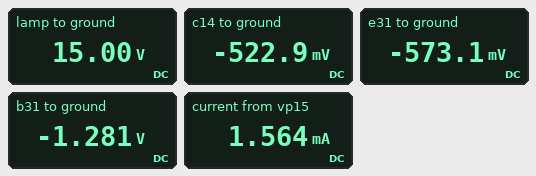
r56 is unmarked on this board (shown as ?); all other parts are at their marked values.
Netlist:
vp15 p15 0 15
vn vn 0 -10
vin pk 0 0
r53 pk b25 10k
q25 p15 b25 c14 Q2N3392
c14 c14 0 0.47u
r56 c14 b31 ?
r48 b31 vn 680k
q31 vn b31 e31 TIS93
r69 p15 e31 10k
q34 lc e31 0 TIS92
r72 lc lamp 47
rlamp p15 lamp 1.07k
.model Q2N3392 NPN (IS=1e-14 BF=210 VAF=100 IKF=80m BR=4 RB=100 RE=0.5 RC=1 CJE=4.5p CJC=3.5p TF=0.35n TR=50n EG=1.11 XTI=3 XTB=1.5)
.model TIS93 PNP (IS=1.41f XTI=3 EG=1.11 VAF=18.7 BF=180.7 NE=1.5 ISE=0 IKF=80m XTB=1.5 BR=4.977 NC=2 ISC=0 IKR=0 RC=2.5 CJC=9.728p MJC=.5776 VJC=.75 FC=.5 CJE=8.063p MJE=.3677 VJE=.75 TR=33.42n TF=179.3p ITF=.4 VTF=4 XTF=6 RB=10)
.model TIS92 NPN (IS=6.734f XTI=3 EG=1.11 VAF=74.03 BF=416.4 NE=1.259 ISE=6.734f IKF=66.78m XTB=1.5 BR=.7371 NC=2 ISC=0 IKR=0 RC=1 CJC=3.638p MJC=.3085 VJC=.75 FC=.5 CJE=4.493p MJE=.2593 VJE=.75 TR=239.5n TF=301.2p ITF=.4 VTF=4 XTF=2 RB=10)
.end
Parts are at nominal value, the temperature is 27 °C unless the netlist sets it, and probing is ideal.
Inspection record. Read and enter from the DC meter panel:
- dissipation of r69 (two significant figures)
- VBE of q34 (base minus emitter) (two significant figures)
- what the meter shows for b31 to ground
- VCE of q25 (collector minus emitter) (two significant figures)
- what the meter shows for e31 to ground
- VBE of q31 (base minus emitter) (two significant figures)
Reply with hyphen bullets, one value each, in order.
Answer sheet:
- 24 mW
- -570 mV
- -1.281 V
- 16 V
- -573.1 mV
- -710 mV
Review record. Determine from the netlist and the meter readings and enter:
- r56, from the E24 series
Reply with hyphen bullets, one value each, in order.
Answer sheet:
- 110 kΩ
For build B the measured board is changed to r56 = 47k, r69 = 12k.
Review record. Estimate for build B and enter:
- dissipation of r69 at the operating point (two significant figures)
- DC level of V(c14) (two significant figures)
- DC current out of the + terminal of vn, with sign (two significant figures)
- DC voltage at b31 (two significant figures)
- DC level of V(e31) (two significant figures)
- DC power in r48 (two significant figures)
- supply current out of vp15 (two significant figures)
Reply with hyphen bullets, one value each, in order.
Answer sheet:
- 19 mW
- -530 mV
- -1.3 mA
- -930 mV
- -230 mV
- 120 µW
- 1.3 mA
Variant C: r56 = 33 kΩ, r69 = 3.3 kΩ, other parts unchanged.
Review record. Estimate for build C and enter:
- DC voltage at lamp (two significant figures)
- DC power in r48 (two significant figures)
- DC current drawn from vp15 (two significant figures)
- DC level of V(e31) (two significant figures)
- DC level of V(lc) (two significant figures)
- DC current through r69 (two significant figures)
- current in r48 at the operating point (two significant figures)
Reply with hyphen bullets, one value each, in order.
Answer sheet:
- 750 mV
- 150 µW
- 18 mA
- 740 mV
- 130 mV
- 4.3 mA
- 15 µA
